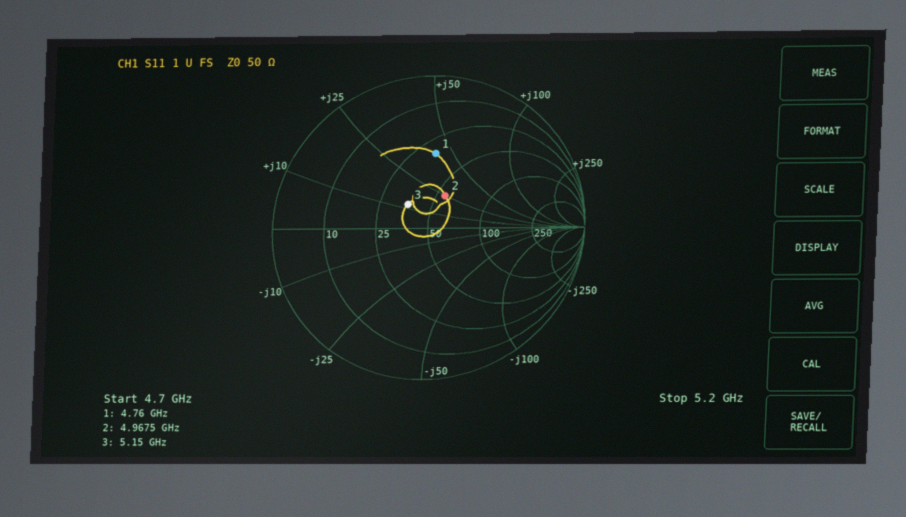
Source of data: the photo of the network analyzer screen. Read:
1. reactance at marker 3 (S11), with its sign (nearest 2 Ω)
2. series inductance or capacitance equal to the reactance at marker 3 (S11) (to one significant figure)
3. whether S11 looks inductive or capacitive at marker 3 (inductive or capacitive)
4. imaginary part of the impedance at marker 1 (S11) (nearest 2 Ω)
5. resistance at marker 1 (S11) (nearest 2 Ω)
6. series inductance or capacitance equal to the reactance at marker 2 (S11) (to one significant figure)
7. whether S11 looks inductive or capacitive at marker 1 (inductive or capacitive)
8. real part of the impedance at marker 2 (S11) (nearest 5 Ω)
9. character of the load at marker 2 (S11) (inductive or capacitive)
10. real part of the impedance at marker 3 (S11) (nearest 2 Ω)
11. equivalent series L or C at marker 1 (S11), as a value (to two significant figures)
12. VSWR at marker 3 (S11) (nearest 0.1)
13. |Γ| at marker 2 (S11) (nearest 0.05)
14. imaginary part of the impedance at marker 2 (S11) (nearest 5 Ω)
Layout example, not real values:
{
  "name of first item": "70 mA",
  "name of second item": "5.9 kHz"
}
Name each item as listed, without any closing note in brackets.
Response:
{
  "reactance at marker 3 (S11), with its sign": "+12 Ω",
  "series inductance or capacitance equal to the reactance at marker 3 (S11)": "400 pH",
  "whether S11 looks inductive or capacitive at marker 3": "inductive",
  "imaginary part of the impedance at marker 1 (S11)": "+42 Ω",
  "resistance at marker 1 (S11)": "32 Ω",
  "series inductance or capacitance equal to the reactance at marker 2 (S11)": "800 pH",
  "whether S11 looks inductive or capacitive at marker 1": "inductive",
  "real part of the impedance at marker 2 (S11)": "55 Ω",
  "character of the load at marker 2 (S11)": "inductive",
  "real part of the impedance at marker 3 (S11)": "36 Ω",
  "equivalent series L or C at marker 1 (S11), as a value": "1.4 nH",
  "VSWR at marker 3 (S11)": "1.5",
  "|Γ| at marker 2 (S11)": "0.25",
  "imaginary part of the impedance at marker 2 (S11)": "+25 Ω"
}
